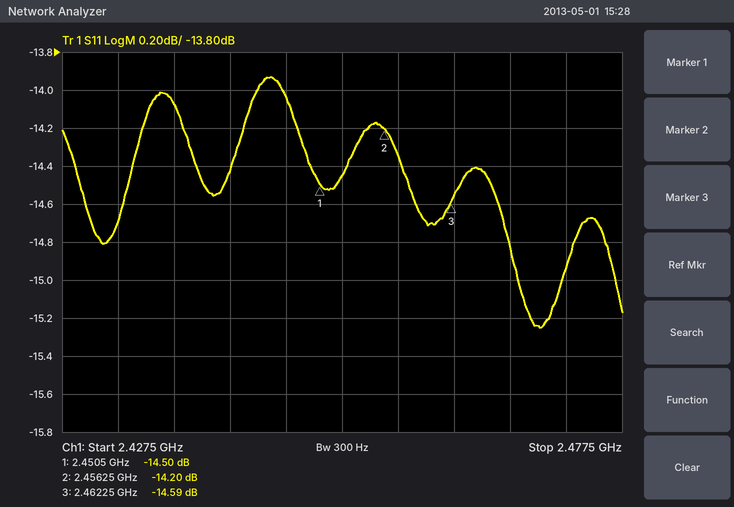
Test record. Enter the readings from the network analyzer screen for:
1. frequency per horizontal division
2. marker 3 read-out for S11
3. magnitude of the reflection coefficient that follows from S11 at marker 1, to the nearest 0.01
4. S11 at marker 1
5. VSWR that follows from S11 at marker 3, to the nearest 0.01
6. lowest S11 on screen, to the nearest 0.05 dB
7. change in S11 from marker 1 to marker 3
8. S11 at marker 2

5 MHz
-14.59 dB
0.19
-14.50 dB
1.46
-15.25 dB
-0.09 dB
-14.20 dB
